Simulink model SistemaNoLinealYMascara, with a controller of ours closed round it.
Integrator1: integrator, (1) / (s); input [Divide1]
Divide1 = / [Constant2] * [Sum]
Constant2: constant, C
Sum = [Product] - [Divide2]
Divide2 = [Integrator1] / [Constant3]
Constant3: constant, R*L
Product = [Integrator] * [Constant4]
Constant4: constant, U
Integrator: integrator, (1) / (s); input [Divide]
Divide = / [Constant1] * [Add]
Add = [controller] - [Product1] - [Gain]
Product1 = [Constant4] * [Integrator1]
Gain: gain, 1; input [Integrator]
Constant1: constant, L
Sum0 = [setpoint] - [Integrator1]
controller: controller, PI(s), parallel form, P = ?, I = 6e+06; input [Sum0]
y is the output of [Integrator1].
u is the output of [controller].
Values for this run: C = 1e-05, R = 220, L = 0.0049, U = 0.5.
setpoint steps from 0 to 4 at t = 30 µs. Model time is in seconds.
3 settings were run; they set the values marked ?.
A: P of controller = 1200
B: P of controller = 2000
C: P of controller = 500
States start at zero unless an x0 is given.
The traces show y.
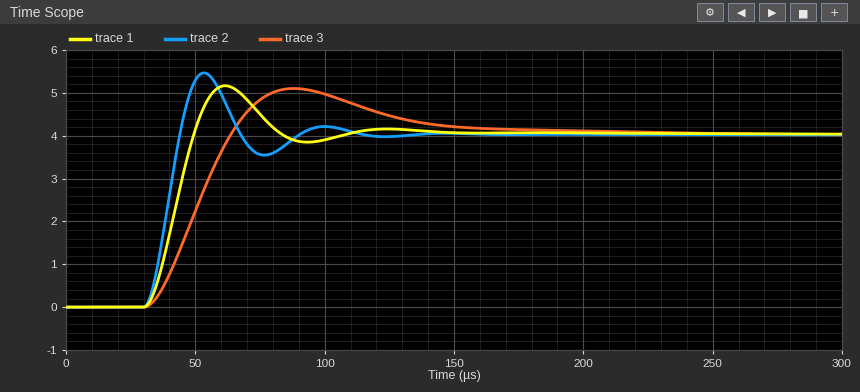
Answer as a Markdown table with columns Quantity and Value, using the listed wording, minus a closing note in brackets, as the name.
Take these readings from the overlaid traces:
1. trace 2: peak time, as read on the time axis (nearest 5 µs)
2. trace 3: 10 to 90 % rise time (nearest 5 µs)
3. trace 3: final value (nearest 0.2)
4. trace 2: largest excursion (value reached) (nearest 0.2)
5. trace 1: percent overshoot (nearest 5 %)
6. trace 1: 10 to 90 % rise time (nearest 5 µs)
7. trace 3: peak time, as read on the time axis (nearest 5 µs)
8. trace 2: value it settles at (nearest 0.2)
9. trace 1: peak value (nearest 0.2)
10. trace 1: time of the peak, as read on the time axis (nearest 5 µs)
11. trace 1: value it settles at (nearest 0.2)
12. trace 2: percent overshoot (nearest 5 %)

| Quantity | Value |
|---|---|
| trace 2: peak time, as read on the time axis | 55 µs |
| trace 3: 10 to 90 % rise time | 25 µs |
| trace 3: final value | 4.0 |
| trace 2: largest excursion (value reached) | 5.4 |
| trace 1: percent overshoot | 30 % |
| trace 1: 10 to 90 % rise time | 15 µs |
| trace 3: peak time, as read on the time axis | 90 µs |
| trace 2: value it settles at | 4.0 |
| trace 1: peak value | 5.2 |
| trace 1: time of the peak, as read on the time axis | 60 µs |
| trace 1: value it settles at | 4.0 |
| trace 2: percent overshoot | 35 % |
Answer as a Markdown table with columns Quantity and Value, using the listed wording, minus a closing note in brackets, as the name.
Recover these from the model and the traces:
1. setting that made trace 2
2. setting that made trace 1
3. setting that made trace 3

| Quantity | Value |
|---|---|
| setting that made trace 2 | B |
| setting that made trace 1 | A |
| setting that made trace 3 | C |
